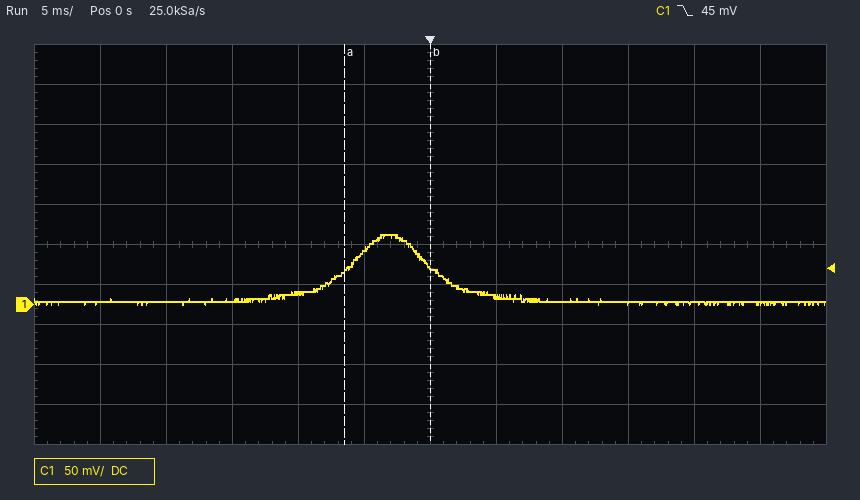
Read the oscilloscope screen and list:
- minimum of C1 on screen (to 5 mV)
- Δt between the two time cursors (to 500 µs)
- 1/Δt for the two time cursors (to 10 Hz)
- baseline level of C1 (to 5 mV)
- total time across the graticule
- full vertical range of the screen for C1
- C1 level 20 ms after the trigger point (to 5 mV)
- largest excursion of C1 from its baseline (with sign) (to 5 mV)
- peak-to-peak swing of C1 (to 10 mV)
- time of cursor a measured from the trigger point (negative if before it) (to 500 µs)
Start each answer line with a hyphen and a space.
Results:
- 0 mV
- 6.5 ms
- 150 Hz
- 5 mV
- 60 ms
- 500 mV
- 5 mV
- +85 mV
- 90 mV
- -6.5 ms
